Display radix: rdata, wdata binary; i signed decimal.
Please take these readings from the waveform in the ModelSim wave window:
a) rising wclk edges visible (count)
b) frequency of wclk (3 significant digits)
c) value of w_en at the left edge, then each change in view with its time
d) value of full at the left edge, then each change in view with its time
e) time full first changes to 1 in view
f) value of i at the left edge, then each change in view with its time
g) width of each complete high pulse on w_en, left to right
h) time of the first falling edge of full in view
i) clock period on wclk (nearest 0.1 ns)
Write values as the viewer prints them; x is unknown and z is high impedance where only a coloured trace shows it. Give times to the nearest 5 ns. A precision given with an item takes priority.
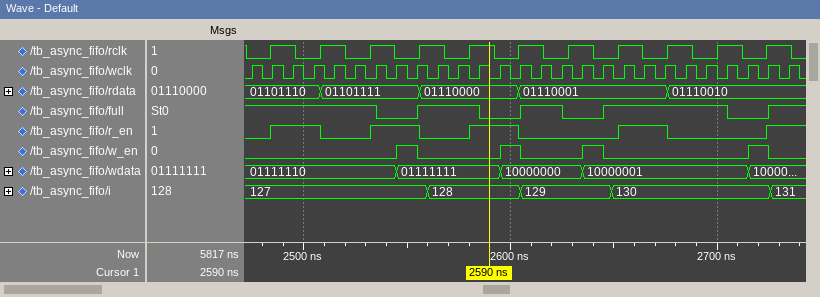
27
100 MHz
0, 1 at 2545 ns, 0 at 2555 ns, 1 at 2595 ns, 0 at 2605 ns, 1 at 2635 ns, 0 at 2645 ns, 1 at 2715 ns, 0 at 2725 ns
1, 0 at 2535 ns, 1 at 2555 ns, 0 at 2585 ns, 1 at 2605 ns, 0 at 2625 ns, 1 at 2645 ns, 0 at 2705 ns, 1 at 2725 ns
2555 ns
127, 128 at 2560 ns, 129 at 2605 ns, 130 at 2650 ns, 131 at 2725 ns
10 ns, 10 ns, 10 ns, 10 ns
2535 ns
10 ns
